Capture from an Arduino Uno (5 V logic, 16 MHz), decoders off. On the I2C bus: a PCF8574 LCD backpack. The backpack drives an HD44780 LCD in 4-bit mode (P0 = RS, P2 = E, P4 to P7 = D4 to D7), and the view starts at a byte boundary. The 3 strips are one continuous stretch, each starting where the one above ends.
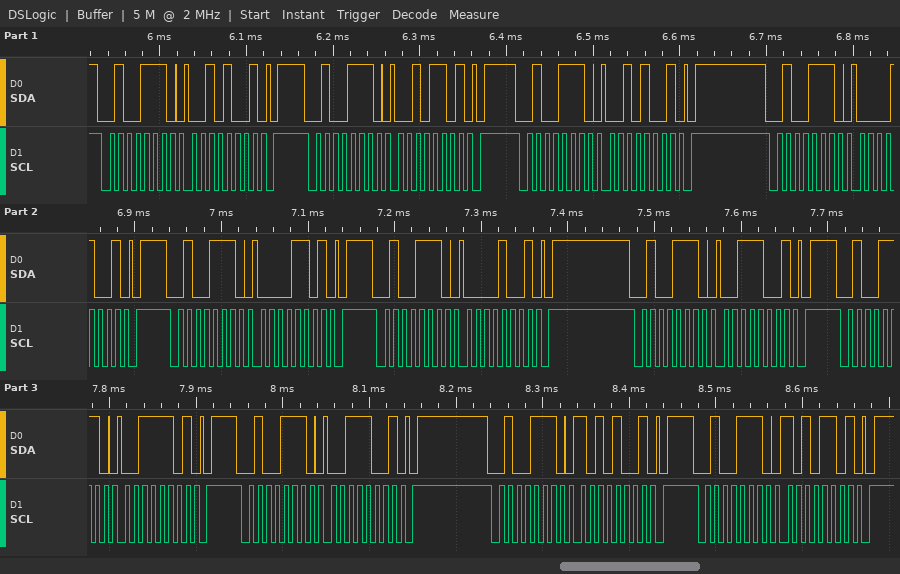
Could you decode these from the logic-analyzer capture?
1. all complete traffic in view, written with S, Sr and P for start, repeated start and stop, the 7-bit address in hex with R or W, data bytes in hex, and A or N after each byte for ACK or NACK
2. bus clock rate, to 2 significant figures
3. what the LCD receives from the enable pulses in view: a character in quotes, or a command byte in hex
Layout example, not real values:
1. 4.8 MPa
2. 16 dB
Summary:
1. S 27W A 29 A P S 27W A 2D A P S 27W A 29 A P S 27W A 09 A P S 27W A 0D A P S 27W A 09 A P S 27W A 39 A P S 27W A 3D A P S 27W A 39 A P S 27W A A9 A P S 27W A AD A P
2. 100 kHz
3. ' '
